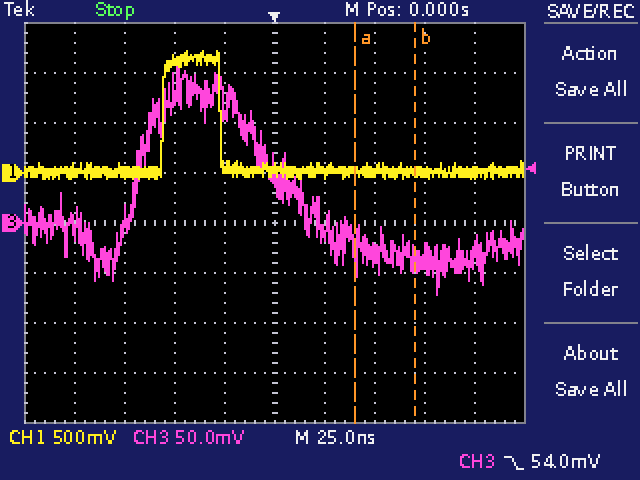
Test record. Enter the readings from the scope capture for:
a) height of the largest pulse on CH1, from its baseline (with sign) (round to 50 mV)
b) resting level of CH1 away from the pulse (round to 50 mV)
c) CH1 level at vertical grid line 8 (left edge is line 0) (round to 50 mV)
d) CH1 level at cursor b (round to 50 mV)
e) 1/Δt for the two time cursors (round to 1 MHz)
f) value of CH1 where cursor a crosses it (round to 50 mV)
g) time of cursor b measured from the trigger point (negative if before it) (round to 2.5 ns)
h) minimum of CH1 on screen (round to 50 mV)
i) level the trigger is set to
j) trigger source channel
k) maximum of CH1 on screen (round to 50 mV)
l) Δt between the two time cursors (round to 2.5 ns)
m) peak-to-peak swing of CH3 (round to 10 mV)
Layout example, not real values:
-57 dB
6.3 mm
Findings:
+1.20 V
0 mV
0 mV
0 mV
33 MHz
0 mV
+70.0 ns
-50 mV
54.0 mV
CH3
1.20 V
30.0 ns
230 mV
